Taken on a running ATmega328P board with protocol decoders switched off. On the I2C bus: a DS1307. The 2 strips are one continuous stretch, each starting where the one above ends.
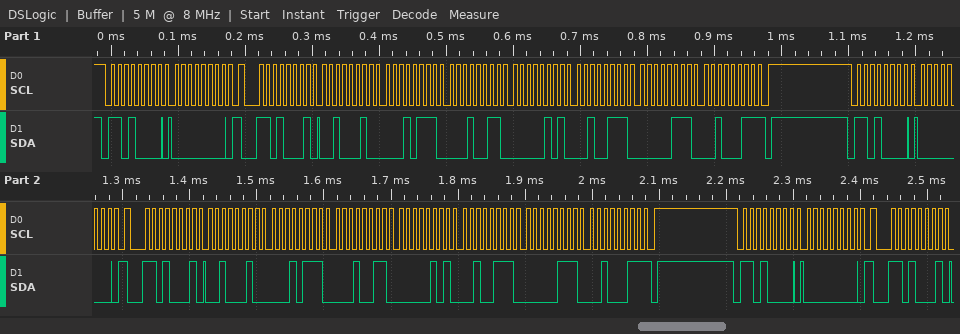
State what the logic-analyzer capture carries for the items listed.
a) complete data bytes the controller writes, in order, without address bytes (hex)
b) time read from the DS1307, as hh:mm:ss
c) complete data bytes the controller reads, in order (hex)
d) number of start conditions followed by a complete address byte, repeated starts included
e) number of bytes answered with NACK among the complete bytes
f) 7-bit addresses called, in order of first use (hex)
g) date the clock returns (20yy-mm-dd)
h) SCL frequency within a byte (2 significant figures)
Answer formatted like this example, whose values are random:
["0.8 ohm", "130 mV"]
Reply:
["00 00 00", "13:17:22", "22 17 13 05 27 07 23 22 17 13 05 27 07 23", "6", "2", "0x68", "2023-07-27", "100 kHz"]
